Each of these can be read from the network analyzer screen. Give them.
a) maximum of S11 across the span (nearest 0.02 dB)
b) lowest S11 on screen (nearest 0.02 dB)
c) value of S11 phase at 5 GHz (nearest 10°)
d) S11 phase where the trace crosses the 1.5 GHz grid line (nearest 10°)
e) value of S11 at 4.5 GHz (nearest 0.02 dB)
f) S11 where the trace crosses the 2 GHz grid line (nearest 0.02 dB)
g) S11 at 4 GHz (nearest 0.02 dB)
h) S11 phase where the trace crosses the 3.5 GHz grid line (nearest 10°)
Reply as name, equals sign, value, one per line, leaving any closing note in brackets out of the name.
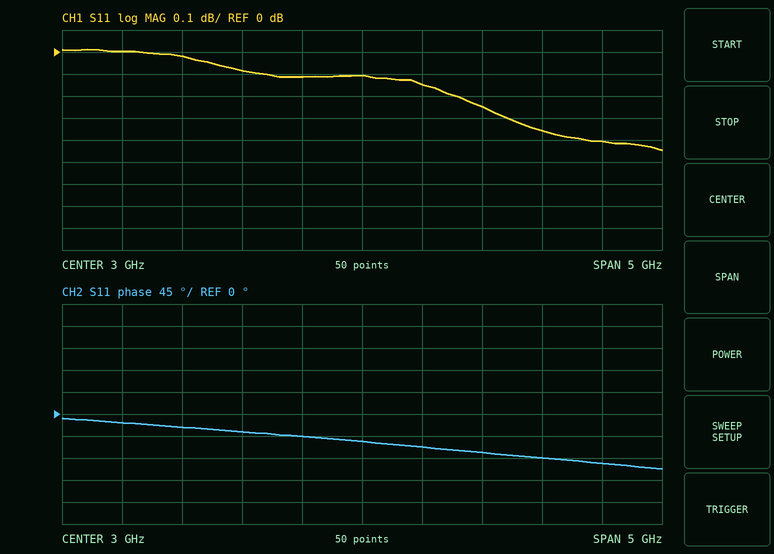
maximum of S11 across the span = 0.02 dB
lowest S11 on screen = -0.44 dB
value of S11 phase at 5 GHz = -100°
S11 phase where the trace crosses the 1.5 GHz grid line = -30°
value of S11 at 4.5 GHz = -0.36 dB
S11 where the trace crosses the 2 GHz grid line = -0.08 dB
S11 at 4 GHz = -0.24 dB
S11 phase where the trace crosses the 3.5 GHz grid line = -70°
